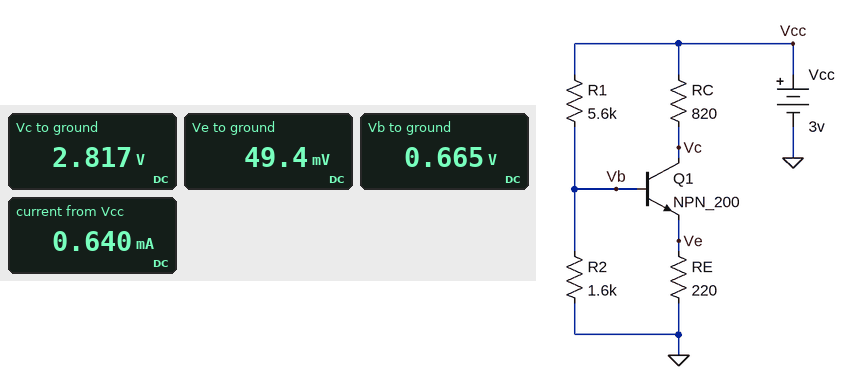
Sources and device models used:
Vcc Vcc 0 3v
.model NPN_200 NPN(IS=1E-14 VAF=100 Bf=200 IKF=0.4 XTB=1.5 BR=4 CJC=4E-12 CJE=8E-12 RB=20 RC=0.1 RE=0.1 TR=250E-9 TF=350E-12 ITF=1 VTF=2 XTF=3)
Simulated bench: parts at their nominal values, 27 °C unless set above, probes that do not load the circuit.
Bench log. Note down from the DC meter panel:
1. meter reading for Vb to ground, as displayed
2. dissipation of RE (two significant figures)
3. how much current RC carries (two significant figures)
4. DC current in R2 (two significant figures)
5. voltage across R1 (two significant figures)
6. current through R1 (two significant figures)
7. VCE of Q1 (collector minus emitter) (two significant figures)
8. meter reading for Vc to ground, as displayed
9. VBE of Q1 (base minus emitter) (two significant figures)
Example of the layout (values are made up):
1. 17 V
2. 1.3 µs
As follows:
1. 0.665 V
2. 11 µW
3. 220 µA
4. 420 µA
5. 2.3 V
6. 420 µA
7. 2.8 V
8. 2.817 V
9. 620 mV
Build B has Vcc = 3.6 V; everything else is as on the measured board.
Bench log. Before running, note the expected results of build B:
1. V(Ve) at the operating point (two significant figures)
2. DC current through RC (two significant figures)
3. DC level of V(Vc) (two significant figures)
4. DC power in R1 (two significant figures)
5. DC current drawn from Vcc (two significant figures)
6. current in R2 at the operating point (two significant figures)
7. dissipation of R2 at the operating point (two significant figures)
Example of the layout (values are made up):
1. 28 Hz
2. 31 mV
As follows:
1. 150 mV
2. 680 µA
3. 3.0 V
4. 1.4 mW
5. 1.2 mA
6. 500 µA
7. 400 µW
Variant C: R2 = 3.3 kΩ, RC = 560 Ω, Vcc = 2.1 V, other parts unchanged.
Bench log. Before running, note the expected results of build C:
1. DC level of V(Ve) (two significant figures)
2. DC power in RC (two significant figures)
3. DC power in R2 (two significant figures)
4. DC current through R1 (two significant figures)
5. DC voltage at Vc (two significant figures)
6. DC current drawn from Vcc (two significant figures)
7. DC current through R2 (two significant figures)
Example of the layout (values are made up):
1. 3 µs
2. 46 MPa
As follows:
1. 130 mV
2. 200 µW
3. 180 µW
4. 240 µA
5. 1.8 V
6. 830 µA
7. 230 µA
